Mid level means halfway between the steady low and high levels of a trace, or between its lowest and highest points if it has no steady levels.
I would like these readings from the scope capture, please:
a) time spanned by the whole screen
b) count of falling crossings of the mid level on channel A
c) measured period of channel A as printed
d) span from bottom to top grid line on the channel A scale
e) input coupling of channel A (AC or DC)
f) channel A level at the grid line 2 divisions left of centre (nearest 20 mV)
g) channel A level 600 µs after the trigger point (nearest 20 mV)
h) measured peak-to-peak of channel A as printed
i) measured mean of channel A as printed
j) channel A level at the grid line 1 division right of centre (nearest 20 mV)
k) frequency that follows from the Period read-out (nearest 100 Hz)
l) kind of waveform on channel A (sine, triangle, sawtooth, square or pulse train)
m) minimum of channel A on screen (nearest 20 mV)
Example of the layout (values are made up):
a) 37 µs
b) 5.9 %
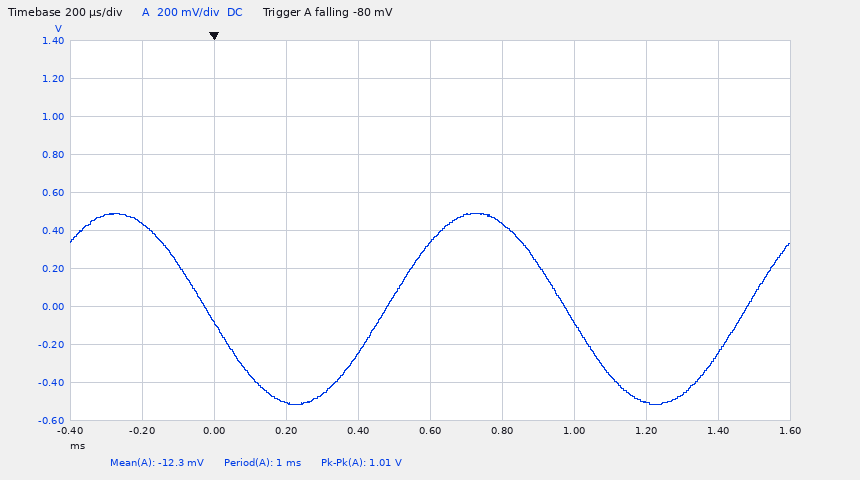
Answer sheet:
a) 2 ms
b) 2
c) 1 ms
d) 2 V
e) DC
f) -500 mV
g) 340 mV
h) 1.01 V
i) -12.3 mV
j) 440 mV
k) 1.0 kHz
l) sine
m) -520 mV
